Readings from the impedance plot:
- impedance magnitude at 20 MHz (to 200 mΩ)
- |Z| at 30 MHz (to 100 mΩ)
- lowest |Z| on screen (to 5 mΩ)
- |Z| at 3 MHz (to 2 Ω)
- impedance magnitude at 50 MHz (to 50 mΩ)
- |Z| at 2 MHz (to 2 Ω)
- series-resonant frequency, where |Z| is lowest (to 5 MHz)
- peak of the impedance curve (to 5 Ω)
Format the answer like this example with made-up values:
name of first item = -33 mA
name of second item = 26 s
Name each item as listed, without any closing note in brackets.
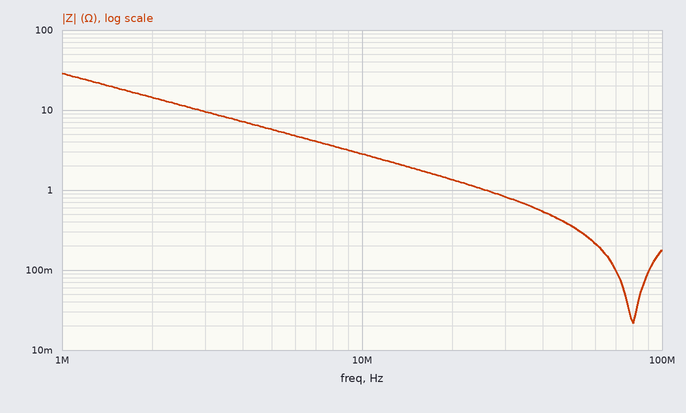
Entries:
impedance magnitude at 20 MHz = 1.4 Ω
|Z| at 30 MHz = 800 mΩ
lowest |Z| on screen = 20 mΩ
|Z| at 3 MHz = 10 Ω
impedance magnitude at 50 MHz = 350 mΩ
|Z| at 2 MHz = 14 Ω
series-resonant frequency, where |Z| is lowest = 80 MHz
peak of the impedance curve = 30 Ω
